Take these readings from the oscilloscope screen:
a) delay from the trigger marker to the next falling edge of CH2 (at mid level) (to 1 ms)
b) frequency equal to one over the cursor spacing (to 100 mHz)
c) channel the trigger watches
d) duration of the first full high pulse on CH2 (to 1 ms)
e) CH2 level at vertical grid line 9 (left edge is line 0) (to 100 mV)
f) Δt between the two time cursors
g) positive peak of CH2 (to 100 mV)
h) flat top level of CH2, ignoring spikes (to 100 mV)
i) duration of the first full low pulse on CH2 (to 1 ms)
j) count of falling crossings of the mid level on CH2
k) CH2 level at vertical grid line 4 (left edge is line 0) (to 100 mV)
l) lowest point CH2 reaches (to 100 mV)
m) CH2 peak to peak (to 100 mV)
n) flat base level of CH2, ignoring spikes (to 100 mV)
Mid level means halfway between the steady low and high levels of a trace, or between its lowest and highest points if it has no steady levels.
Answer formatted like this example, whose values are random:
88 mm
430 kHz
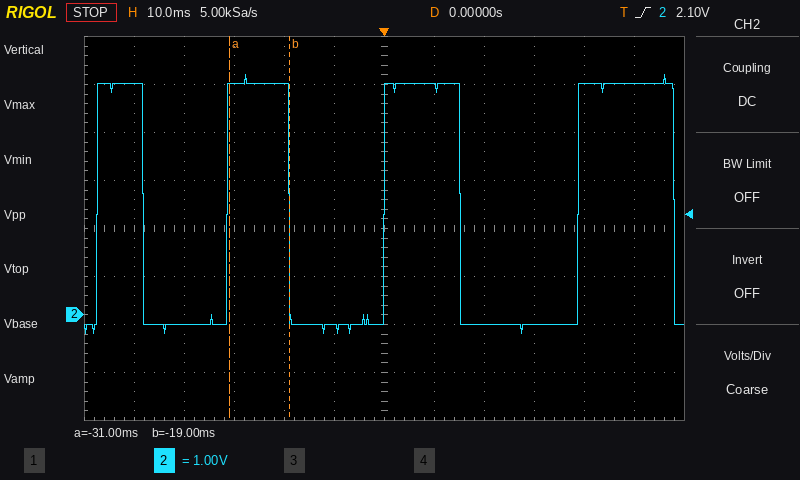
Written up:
15 ms
83.3 Hz
CH2
9 ms
-200 mV
12 ms
5.0 V
4.8 V
17 ms
4
4.8 V
-400 mV
5.4 V
-200 mV
